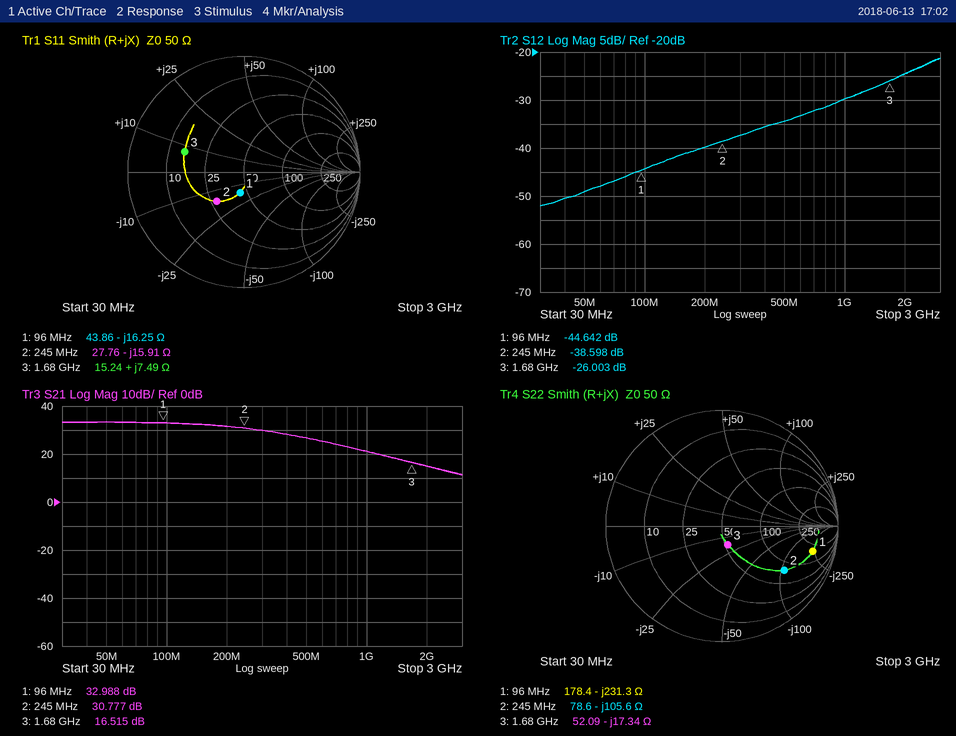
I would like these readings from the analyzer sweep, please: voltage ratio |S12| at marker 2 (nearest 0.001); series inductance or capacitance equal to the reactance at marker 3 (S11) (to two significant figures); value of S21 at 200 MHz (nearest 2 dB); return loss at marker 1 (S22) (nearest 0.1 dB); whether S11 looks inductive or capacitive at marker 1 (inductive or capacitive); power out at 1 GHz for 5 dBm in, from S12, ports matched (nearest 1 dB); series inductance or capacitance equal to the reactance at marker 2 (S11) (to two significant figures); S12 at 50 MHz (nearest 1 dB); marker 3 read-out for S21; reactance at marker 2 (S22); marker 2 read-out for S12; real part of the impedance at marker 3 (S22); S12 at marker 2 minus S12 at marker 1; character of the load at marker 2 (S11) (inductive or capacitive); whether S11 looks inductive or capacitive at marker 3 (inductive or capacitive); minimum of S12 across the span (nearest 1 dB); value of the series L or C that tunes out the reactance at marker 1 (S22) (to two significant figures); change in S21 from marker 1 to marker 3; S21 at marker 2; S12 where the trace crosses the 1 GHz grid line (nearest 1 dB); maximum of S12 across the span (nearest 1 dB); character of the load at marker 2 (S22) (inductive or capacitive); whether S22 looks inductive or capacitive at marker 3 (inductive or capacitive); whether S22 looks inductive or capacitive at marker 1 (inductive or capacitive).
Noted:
0.012
710 pH
32 dB
1.8 dB
capacitive
-25 dBm
41 pF
-49 dB
16.515 dB
-105.6 Ω
-38.598 dB
52.09 Ω
6.044 dB
capacitive
inductive
-52 dB
380 nH
-16.473 dB
30.777 dB
-30 dB
-21 dB
capacitive
capacitive
capacitive
